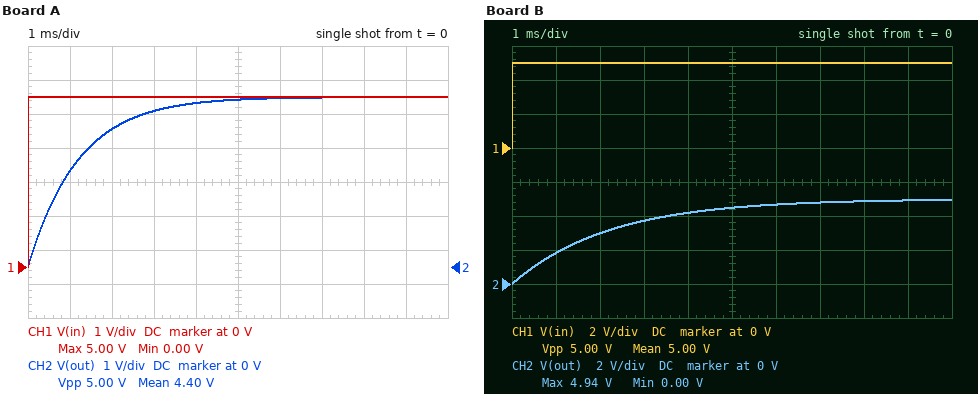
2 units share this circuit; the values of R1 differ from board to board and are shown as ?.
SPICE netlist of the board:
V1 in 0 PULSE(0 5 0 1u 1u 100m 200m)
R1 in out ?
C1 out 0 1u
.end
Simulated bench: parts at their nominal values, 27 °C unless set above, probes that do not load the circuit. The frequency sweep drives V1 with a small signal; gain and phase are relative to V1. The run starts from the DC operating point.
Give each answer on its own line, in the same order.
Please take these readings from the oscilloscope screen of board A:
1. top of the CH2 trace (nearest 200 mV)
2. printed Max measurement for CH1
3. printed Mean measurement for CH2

5.0 V
5.00 V
4.40 V
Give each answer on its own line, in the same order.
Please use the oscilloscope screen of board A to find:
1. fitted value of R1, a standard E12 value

1.2 kΩ
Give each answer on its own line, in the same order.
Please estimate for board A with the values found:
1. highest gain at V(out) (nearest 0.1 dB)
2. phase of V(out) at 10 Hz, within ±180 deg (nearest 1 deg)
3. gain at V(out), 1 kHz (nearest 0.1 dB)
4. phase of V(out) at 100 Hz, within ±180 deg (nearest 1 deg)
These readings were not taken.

0 dB
-4 deg
-17.6 dB
-37 deg
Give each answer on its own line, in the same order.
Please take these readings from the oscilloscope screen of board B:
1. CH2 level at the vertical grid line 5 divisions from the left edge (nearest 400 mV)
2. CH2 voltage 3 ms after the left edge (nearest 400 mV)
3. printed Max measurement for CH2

4.4 V
3.6 V
4.94 V
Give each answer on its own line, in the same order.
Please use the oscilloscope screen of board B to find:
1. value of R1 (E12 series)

2.2 kΩ
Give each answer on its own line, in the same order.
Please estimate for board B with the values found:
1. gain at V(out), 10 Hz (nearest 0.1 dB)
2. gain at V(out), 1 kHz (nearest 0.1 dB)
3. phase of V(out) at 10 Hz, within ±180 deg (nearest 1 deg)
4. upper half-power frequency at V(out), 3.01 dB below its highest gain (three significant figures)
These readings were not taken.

-0.1 dB
-22.8 dB
-8 deg
72.3 Hz
